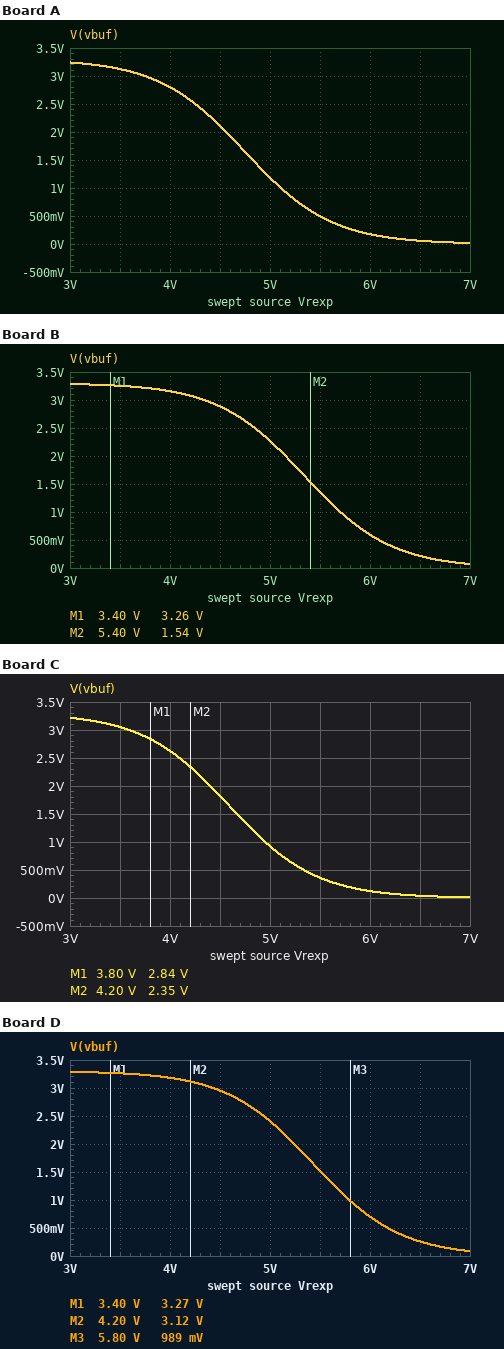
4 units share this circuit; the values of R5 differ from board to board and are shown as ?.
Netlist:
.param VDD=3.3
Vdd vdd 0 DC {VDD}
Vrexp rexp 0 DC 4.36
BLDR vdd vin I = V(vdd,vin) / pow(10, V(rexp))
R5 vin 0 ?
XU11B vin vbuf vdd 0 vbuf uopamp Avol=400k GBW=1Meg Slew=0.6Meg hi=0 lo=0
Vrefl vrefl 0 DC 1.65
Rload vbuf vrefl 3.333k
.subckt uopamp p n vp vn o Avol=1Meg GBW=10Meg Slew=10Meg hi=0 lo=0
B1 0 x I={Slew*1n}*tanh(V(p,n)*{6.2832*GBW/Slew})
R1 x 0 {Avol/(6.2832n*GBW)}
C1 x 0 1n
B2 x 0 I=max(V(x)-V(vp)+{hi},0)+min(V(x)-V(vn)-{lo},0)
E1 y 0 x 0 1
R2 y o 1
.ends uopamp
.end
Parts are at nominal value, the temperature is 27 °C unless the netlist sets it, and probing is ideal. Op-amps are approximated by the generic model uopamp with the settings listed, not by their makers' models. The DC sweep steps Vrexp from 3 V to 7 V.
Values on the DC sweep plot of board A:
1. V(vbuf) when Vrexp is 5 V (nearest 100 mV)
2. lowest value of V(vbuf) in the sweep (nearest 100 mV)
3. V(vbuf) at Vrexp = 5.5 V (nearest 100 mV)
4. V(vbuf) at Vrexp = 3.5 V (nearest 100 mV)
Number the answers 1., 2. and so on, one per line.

1. 1.2 V
2. 0 V
3. 500 mV
4. 3.1 V
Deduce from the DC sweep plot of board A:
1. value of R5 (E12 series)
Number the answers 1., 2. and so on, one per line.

1. 56 kΩ
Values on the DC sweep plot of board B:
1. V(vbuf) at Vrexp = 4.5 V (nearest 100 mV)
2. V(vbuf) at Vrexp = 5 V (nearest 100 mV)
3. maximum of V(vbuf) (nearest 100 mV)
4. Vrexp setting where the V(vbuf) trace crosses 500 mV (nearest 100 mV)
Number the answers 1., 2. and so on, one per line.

1. 2.9 V
2. 2.3 V
3. 3.3 V
4. 6.1 V
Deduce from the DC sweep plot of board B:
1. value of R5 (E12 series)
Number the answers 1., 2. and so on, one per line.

1. 220 kΩ
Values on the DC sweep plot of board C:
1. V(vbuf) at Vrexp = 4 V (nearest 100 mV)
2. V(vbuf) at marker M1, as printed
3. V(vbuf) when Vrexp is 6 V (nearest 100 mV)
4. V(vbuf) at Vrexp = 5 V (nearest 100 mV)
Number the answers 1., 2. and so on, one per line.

1. 2.6 V
2. 2.84 V
3. 100 mV
4. 900 mV
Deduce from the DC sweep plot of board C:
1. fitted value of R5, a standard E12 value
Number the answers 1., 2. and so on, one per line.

1. 39 kΩ
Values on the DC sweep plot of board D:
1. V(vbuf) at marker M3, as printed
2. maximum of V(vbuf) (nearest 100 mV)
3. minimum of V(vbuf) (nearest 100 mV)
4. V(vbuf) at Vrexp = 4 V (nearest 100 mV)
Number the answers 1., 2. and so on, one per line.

1. 989 mV
2. 3.3 V
3. 100 mV
4. 3.2 V
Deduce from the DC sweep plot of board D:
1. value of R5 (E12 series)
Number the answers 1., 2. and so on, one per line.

1. 270 kΩ
